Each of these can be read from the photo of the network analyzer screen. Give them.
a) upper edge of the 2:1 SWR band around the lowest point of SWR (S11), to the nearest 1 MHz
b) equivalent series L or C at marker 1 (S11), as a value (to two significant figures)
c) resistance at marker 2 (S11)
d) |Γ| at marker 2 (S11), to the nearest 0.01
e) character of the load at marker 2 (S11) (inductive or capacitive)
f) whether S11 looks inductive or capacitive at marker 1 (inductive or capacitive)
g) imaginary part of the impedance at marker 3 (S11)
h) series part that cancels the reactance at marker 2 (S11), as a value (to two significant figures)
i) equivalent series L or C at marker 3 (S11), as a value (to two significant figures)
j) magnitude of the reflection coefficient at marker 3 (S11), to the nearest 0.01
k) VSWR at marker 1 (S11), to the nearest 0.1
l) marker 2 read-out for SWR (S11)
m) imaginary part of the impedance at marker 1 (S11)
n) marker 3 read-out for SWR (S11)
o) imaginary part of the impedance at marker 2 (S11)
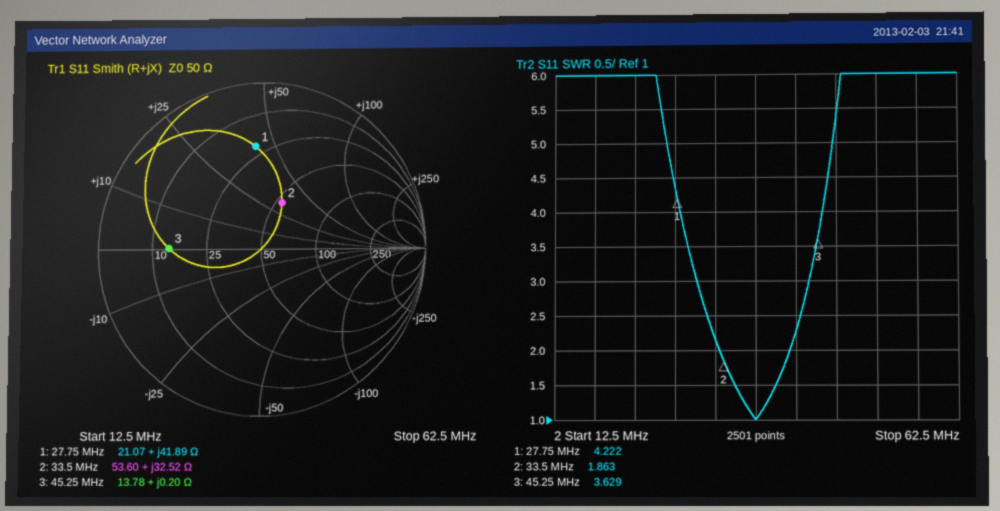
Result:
42 MHz
240 nH
53.60 Ω
0.30
inductive
inductive
+0.20 Ω
150 pF
700 pH
0.57
4.2
1.863
+41.89 Ω
3.629
+32.52 Ω
